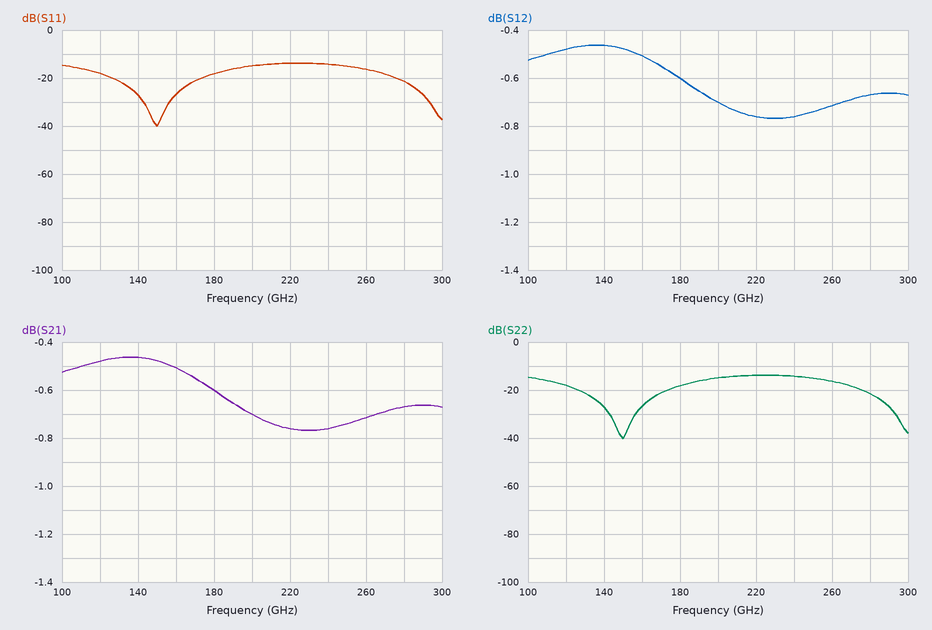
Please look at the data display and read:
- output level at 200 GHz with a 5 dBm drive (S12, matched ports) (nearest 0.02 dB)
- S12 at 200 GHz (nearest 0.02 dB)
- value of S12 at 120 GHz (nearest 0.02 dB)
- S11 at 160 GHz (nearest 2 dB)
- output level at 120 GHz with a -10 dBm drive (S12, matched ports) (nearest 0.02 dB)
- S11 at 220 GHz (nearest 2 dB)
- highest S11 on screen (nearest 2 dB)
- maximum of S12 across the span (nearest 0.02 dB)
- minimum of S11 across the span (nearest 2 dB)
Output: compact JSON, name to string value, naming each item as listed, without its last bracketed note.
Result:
{"output level at 200 GHz with a 5 dBm drive (S12, matched ports)": "4.30 dBm", "S12 at 200 GHz": "-0.70 dB", "value of S12 at 120 GHz": "-0.48 dB", "S11 at 160 GHz": "-26 dB", "output level at 120 GHz with a -10 dBm drive (S12, matched ports)": "-10.48 dBm", "S11 at 220 GHz": "-14 dB", "highest S11 on screen": "-14 dB", "maximum of S12 across the span": "-0.46 dB", "minimum of S11 across the span": "-40 dB"}
